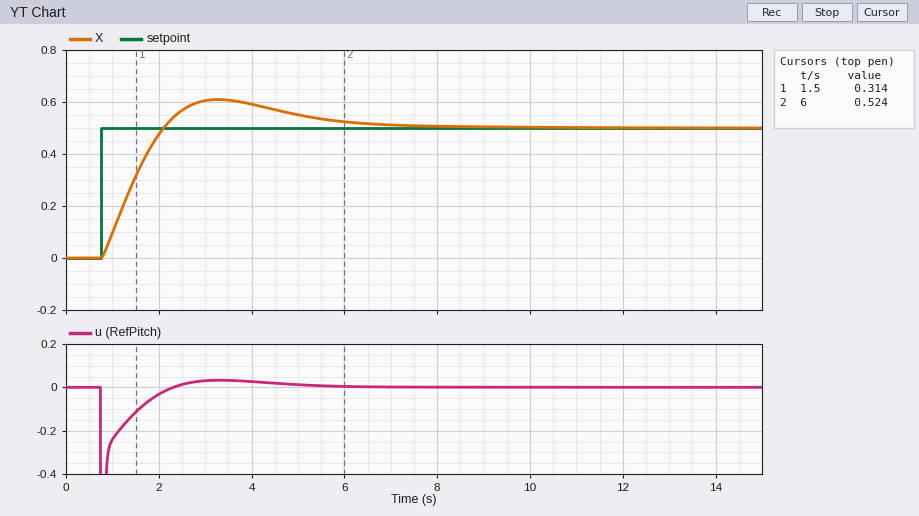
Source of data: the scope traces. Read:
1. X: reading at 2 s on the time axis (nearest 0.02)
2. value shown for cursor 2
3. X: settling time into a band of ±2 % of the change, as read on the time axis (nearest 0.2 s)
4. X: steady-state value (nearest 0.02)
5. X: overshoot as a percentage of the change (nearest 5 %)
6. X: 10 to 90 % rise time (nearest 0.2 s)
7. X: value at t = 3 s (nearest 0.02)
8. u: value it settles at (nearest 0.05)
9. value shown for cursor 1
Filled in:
0.48
0.524
7.2 s
0.50
20 %
1.0 s
0.60
0.00
0.314
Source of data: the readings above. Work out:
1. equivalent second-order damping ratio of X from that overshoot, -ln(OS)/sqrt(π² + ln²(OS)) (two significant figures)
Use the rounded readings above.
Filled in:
0.46
